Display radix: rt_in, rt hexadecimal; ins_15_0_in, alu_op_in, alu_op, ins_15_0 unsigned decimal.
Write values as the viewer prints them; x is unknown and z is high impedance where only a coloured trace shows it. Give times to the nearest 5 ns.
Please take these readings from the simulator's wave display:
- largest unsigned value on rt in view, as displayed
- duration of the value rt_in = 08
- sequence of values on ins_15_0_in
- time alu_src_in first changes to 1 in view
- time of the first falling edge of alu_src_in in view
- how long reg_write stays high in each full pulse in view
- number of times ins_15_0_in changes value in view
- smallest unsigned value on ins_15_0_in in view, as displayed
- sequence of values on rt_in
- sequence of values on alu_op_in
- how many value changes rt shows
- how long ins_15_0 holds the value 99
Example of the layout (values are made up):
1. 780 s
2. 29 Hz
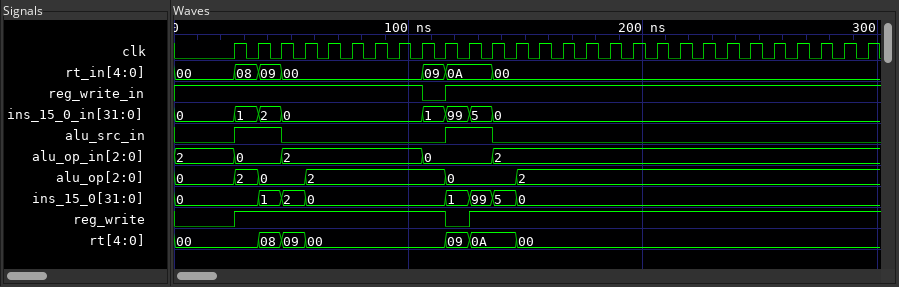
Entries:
1. 0A
2. 10 ns
3. 0, 1, 2, 0, 1, 99, 5, 0
4. 25 ns
5. 45 ns
6. 90 ns
7. 7
8. 0
9. 00, 08, 09, 00, 09, 0A, 00
10. 2, 0, 2, 0, 2
11. 6
12. 10 ns
